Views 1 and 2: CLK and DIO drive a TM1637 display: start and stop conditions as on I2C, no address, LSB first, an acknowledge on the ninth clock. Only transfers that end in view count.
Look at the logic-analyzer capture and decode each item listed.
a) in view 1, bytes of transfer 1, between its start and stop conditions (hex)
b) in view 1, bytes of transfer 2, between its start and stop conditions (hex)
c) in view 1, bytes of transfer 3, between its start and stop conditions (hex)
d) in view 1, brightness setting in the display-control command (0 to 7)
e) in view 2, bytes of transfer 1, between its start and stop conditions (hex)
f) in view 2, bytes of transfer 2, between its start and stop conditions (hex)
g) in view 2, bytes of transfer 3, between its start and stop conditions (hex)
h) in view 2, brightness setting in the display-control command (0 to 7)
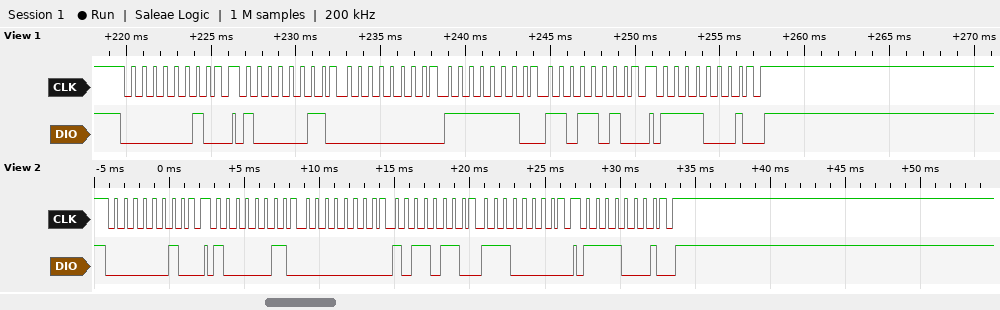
40
C1 00 7F 5B
8F
7
40
C1 00 6D 07
8F
7
